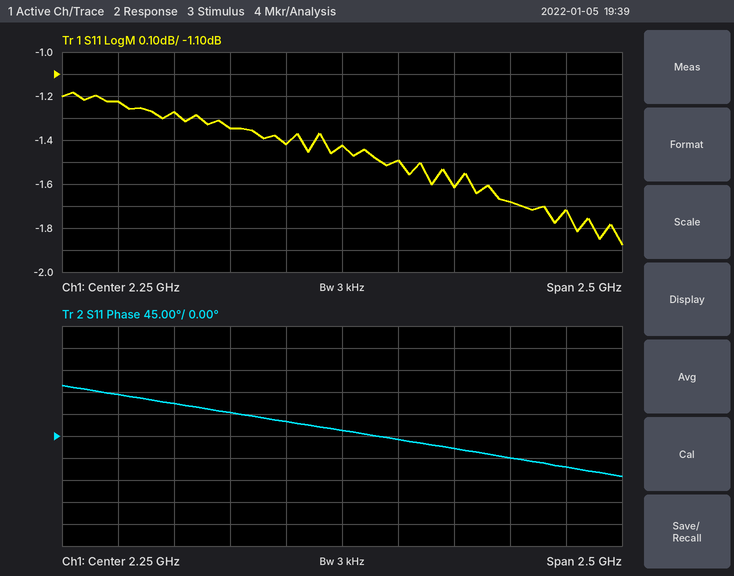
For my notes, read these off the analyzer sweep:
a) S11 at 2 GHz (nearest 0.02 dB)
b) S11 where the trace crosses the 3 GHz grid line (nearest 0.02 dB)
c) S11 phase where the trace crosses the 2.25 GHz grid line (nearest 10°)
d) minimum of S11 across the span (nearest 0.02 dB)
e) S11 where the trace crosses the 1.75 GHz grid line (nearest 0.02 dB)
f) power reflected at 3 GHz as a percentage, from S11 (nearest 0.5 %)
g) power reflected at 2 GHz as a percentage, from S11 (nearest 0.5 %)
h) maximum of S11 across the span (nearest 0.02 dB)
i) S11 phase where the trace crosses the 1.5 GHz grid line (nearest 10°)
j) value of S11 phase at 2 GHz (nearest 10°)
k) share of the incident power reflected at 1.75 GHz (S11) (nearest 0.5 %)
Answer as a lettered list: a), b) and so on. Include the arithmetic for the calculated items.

a) -1.42 dB
b) -1.68 dB
c) 10°
d) -1.88 dB
e) -1.34 dB
f) 10^(-1.68/10) ≈ 67.9 %, so 68.0 % to the nearest 0.5 %
g) 10^(-1.42/10) ≈ 72.1 %, so 72.0 % to the nearest 0.5 %
h) -1.18 dB
i) 70°
j) 30°
k) 10^(-1.34/10) ≈ 73.5 %
